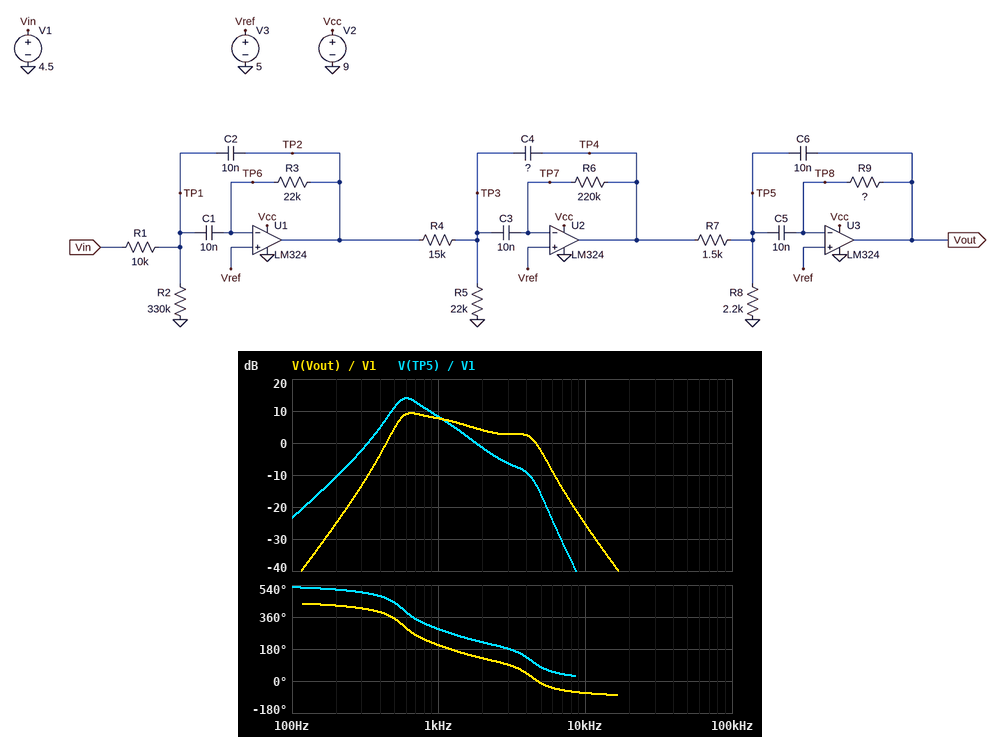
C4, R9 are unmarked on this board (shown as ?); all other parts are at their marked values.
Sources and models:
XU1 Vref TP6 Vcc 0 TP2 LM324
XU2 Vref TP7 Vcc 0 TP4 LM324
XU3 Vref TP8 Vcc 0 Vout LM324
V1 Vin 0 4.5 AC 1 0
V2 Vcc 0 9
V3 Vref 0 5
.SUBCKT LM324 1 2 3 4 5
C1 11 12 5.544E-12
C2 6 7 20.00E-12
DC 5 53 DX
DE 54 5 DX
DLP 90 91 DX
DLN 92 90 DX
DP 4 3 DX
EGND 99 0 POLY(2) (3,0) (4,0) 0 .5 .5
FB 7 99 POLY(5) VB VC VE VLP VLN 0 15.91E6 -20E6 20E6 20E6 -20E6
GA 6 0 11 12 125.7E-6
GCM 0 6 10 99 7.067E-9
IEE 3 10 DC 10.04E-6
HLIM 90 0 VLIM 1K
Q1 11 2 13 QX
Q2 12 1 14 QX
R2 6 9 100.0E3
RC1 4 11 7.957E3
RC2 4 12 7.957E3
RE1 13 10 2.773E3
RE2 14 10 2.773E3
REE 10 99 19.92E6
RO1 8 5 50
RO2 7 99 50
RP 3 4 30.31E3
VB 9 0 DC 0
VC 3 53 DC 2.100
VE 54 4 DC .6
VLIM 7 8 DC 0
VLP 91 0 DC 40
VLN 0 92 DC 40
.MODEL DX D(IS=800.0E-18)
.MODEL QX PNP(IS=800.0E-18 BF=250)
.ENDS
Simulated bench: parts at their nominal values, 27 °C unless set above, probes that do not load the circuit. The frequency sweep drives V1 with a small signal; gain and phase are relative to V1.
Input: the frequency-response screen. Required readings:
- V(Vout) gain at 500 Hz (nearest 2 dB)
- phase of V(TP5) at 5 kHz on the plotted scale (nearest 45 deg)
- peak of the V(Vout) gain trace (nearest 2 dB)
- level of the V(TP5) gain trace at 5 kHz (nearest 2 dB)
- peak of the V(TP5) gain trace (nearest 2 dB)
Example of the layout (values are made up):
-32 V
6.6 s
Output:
4 dB
90 deg
10 dB
-16 dB
14 dB
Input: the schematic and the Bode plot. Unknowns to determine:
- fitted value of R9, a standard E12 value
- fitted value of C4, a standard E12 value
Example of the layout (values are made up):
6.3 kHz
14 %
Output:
15 kΩ
3.9 nF
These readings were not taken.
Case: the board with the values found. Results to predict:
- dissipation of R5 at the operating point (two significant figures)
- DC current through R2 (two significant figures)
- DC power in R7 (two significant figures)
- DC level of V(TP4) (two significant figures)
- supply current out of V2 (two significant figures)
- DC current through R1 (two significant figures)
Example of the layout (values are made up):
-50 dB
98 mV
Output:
400 µW
13 µA
2.7 mW
5.0 V
920 µA
13 µA
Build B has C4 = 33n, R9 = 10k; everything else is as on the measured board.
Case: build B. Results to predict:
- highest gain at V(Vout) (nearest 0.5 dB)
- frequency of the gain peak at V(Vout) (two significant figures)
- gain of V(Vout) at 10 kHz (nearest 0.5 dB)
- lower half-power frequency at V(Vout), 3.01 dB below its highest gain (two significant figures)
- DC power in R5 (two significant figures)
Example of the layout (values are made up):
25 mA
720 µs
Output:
-17.0 dB
1.1 kHz
-43.5 dB
540 Hz
400 µW
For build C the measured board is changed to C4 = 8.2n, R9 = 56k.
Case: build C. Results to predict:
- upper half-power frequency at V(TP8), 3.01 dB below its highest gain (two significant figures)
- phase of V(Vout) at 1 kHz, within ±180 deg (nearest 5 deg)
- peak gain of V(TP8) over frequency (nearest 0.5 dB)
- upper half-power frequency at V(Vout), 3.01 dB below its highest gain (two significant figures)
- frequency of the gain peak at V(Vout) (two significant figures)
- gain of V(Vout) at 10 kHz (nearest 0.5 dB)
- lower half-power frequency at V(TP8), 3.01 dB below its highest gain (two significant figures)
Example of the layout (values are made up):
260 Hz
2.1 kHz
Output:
2.5 kHz
-170 deg
-35.0 dB
2.4 kHz
2.2 kHz
-33.0 dB
1.9 kHz
